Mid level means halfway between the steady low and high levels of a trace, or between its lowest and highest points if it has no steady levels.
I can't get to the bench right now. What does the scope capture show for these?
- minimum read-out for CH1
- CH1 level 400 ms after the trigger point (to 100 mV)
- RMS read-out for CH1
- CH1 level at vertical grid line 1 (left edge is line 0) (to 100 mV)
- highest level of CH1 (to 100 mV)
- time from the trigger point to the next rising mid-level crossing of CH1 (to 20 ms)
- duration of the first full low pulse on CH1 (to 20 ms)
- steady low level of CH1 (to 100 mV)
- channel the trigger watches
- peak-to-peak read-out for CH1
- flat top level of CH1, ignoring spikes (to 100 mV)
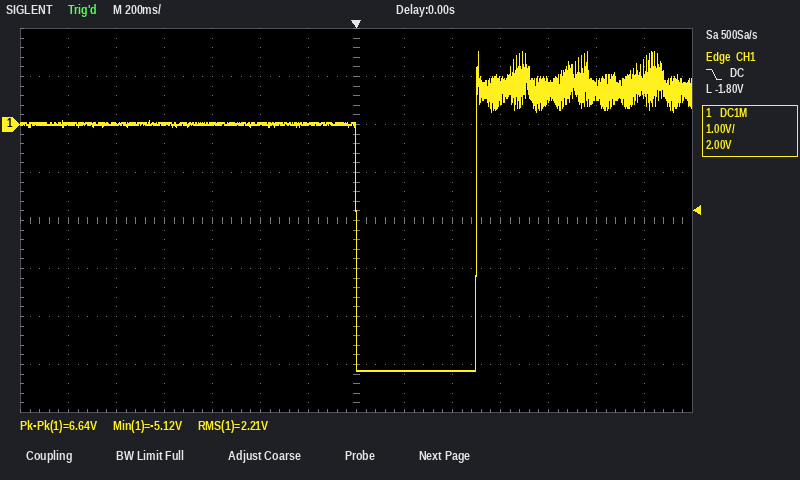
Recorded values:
-5.12 V
-5.1 V
2.21 V
0.0 V
1.5 V
500 ms
500 ms
-5.1 V
CH1
6.64 V
0.0 V
